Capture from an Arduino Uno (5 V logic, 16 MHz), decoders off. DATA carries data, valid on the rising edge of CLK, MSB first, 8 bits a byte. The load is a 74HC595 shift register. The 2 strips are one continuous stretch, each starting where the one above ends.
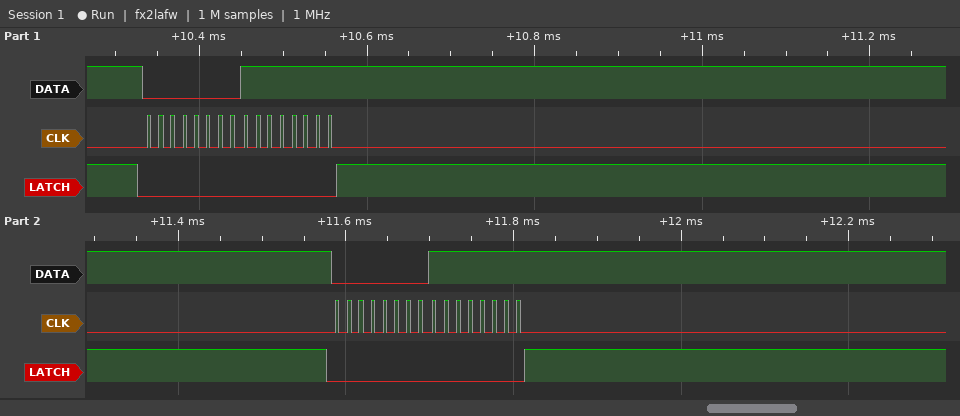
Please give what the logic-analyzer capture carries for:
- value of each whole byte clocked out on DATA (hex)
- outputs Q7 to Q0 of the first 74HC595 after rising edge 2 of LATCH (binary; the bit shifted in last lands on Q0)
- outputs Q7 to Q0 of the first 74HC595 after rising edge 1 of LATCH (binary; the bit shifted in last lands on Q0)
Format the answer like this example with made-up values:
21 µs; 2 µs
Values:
00 FF 00 FF; 11111111; 11111111
